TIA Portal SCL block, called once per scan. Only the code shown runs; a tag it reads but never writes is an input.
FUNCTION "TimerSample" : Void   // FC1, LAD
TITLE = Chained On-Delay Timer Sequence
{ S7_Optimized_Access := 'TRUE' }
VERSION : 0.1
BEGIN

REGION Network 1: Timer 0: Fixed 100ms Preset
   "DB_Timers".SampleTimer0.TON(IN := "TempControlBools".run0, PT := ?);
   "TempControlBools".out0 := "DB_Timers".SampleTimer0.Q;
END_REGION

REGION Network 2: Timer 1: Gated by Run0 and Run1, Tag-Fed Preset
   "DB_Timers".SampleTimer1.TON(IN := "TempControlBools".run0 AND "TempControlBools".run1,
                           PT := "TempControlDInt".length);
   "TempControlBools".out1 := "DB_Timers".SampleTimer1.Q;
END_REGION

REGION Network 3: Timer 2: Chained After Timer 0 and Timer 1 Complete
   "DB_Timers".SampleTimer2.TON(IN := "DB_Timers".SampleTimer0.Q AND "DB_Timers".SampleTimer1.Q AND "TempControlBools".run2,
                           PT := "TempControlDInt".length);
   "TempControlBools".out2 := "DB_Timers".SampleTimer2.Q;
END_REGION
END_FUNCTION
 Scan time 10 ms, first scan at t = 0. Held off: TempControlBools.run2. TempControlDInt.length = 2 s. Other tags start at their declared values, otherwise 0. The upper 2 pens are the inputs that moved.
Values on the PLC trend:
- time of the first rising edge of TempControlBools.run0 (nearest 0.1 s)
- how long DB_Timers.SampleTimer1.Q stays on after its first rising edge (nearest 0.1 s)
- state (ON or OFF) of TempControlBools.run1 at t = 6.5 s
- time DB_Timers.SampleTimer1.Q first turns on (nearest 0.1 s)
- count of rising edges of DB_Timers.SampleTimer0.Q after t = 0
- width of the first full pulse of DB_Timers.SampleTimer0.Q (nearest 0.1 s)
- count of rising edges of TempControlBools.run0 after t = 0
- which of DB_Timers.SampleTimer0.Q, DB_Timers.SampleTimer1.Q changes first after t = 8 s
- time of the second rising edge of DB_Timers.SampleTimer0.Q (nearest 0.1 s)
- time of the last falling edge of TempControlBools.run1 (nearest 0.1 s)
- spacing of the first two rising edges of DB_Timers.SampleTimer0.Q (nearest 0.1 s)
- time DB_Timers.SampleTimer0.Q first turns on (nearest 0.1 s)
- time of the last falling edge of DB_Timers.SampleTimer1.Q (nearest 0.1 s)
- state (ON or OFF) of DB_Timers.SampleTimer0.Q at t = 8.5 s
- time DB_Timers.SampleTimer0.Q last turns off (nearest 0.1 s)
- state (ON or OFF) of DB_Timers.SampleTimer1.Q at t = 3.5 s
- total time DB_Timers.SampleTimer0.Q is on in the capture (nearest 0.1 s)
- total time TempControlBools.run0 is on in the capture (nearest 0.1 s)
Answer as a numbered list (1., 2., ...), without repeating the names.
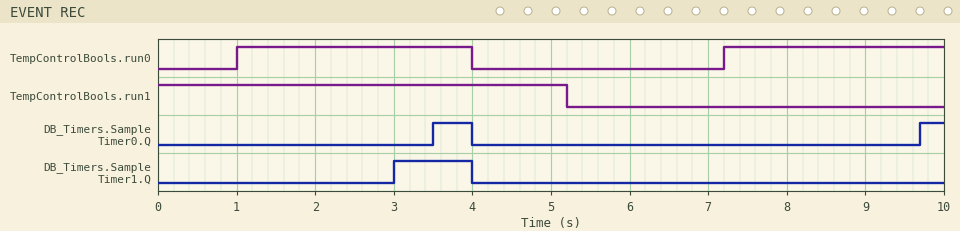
1. 1.0 s
2. 1.0 s
3. OFF
4. 3.0 s
5. 2
6. 0.5 s
7. 2
8. DB_Timers.SampleTimer0.Q
9. 9.7 s
10. 5.2 s
11. 6.2 s
12. 3.5 s
13. 4.0 s
14. OFF
15. 4.0 s
16. ON
17. 0.8 s
18. 5.8 s
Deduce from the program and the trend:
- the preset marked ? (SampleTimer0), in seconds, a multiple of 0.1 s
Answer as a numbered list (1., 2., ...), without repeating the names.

1. 2.5 s
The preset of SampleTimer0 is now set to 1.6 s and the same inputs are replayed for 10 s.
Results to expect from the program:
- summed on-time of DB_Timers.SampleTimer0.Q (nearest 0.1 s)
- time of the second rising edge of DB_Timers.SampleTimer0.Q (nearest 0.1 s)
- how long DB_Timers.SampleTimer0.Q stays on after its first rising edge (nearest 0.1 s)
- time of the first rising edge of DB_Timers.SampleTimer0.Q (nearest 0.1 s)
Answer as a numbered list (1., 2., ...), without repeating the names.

1. 2.6 s
2. 8.8 s
3. 1.4 s
4. 2.6 s
